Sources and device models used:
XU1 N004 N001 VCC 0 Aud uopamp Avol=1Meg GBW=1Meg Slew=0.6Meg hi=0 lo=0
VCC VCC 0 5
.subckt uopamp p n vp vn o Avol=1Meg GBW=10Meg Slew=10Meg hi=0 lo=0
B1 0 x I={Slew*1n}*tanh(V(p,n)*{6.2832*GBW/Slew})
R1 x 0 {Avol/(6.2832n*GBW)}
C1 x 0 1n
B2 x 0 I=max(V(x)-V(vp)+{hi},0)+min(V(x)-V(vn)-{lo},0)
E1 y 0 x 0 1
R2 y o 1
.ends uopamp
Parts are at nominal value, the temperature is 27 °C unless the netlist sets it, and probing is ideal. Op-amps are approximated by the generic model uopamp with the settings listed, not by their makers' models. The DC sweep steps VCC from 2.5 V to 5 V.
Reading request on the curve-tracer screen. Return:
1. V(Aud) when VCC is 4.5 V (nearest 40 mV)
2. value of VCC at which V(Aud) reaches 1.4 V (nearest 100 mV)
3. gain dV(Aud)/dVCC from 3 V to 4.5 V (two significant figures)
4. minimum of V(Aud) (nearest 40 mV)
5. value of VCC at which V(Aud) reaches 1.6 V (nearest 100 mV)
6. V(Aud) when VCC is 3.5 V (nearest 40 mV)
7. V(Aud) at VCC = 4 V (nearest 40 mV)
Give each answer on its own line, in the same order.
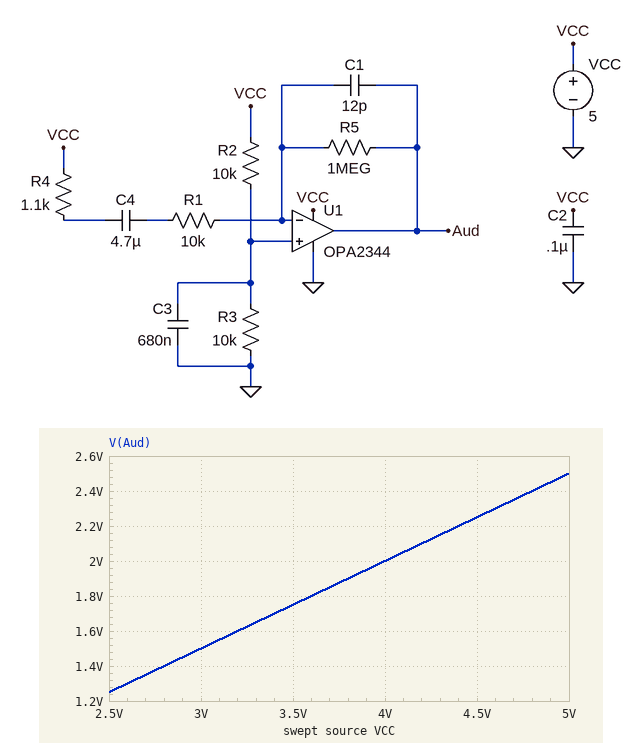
2.24 V
2.8 V
0.50 V/V
1.24 V
3.2 V
1.76 V
2.00 V
